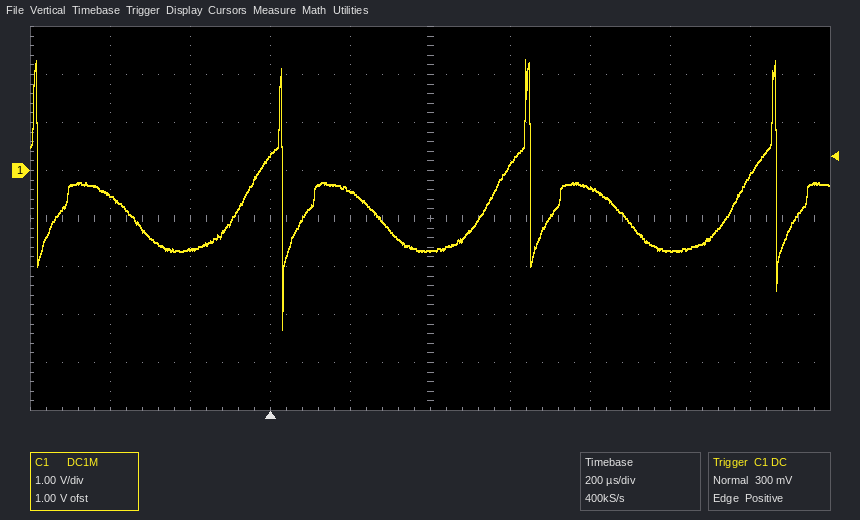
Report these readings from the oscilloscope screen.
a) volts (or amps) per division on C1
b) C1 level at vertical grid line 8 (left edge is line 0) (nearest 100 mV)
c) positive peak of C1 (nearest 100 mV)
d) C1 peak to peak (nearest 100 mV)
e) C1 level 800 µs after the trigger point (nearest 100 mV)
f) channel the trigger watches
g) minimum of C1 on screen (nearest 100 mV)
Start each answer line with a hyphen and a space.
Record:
- 1 V
- -1.7 V
- 2.3 V
- 5.6 V
- -400 mV
- C1
- -3.3 V
